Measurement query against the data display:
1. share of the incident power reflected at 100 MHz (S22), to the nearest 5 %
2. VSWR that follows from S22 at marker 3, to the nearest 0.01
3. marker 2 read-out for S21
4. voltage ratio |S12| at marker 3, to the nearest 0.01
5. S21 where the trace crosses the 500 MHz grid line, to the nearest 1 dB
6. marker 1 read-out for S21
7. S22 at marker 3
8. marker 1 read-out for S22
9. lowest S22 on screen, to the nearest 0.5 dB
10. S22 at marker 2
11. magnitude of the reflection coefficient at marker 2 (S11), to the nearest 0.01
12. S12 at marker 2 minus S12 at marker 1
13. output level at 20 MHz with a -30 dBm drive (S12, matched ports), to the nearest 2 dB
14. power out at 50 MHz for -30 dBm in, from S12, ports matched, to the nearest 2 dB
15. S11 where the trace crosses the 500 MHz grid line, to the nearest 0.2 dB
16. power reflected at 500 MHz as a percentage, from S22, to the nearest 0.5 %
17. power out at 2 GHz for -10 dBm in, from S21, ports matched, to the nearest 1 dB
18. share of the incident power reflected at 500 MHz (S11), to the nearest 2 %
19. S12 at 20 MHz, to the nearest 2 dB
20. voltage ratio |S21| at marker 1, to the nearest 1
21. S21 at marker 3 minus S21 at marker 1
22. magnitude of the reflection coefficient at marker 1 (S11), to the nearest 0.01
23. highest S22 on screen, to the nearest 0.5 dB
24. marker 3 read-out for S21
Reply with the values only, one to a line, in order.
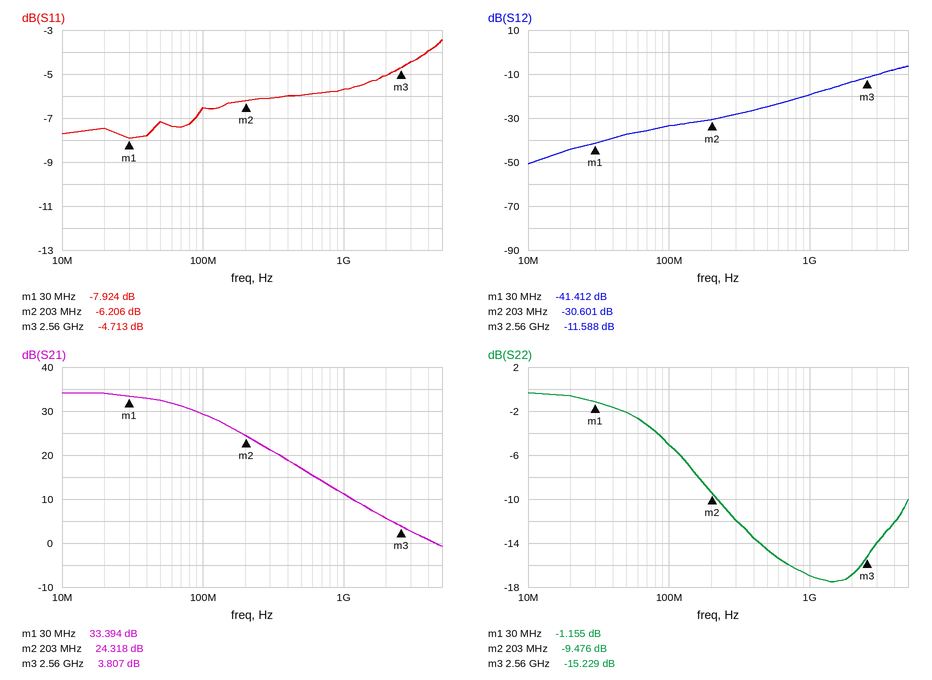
30 %
1.42
24.318 dB
0.26
17 dB
33.394 dB
-15.229 dB
-1.155 dB
-17.5 dB
-9.476 dB
0.49
10.811 dB
-74 dBm
-68 dBm
-6.0 dB
3.5 %
-4 dBm
26 %
-44 dB
47
-29.587 dB
0.40
-0.5 dB
3.807 dB
